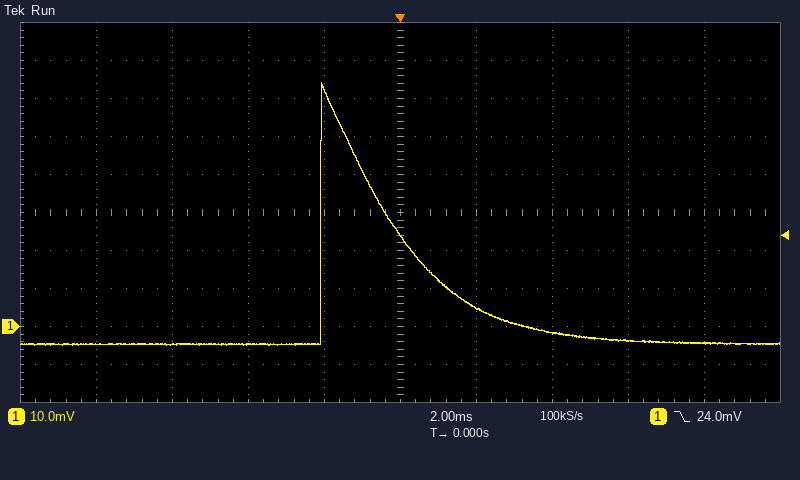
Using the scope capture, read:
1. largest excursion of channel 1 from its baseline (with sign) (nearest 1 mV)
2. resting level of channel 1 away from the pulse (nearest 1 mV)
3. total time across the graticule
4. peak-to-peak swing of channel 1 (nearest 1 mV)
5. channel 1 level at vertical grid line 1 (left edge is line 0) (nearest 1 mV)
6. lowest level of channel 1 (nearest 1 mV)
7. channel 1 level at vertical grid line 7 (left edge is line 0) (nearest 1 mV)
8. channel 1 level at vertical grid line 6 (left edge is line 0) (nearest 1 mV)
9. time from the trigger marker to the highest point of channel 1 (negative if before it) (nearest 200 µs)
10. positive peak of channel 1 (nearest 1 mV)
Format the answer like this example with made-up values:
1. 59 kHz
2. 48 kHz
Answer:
1. +69 mV
2. -5 mV
3. 20 ms
4. 69 mV
5. -5 mV
6. -5 mV
7. -2 mV
8. 5 mV
9. -2.0 ms
10. 64 mV
